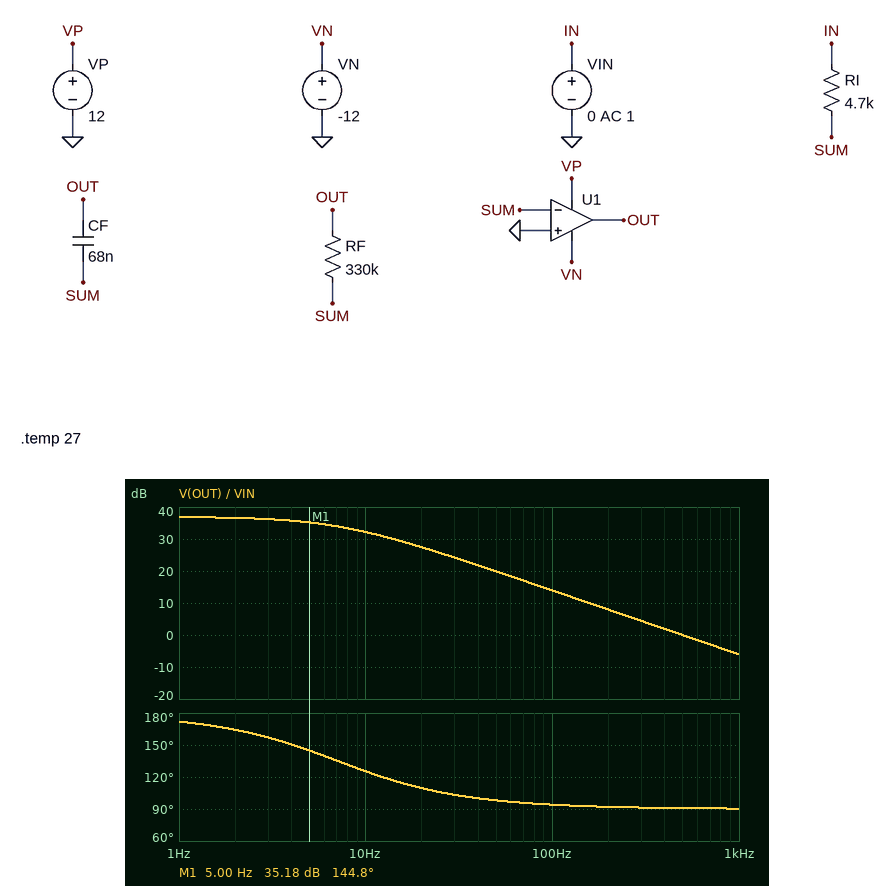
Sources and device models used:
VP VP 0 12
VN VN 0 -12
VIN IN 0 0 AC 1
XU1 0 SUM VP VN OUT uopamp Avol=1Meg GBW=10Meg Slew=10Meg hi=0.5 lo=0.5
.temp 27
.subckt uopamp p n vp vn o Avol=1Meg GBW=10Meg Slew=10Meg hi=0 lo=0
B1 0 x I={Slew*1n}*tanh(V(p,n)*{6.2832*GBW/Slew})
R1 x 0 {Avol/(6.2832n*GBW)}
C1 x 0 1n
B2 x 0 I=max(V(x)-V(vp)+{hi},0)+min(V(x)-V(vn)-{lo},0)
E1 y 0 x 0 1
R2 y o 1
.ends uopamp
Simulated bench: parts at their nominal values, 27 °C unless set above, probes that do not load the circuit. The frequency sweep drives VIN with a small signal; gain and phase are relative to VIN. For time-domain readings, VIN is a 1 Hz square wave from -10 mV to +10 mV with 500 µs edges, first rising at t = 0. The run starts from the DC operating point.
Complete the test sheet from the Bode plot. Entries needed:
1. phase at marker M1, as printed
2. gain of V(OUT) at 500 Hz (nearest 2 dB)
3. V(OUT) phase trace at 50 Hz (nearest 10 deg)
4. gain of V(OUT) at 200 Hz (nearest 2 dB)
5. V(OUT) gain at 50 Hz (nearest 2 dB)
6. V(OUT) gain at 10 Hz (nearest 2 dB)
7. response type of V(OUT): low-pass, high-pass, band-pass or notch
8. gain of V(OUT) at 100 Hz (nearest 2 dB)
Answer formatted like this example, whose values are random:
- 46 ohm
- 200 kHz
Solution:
- 144.8 deg
- 0 dB
- 100 deg
- 8 dB
- 20 dB
- 32 dB
- low-pass
- 14 dB
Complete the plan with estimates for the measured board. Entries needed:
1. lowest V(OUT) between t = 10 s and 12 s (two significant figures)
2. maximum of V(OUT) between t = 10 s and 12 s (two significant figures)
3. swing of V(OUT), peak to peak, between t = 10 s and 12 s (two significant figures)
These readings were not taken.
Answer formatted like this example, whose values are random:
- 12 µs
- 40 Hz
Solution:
- -700 mV
- 700 mV
- 1.4 V
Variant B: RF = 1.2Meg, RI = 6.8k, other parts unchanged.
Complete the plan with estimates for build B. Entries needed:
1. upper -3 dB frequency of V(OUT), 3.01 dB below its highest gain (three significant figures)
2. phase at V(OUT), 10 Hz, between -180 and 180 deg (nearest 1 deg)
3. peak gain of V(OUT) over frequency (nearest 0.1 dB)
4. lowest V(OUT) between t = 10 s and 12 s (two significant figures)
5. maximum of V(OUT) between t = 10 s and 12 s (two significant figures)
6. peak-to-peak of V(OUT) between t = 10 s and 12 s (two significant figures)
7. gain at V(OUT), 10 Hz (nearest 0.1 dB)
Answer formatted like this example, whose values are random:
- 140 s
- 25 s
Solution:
- 1.95 Hz
- 101 deg
- 44.9 dB
- -1.8 V
- 1.8 V
- 3.5 V
- 30.6 dB
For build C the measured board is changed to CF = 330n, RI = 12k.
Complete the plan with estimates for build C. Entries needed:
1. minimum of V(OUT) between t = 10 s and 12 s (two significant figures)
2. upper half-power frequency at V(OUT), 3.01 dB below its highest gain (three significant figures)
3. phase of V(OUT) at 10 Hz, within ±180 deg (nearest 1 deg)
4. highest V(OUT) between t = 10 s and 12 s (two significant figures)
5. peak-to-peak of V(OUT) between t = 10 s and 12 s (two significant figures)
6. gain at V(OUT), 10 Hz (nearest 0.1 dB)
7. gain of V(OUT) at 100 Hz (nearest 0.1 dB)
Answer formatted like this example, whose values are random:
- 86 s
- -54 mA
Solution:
- -270 mV
- 1.46 Hz
- 98 deg
- 270 mV
- 540 mV
- 12.0 dB
- -7.9 dB
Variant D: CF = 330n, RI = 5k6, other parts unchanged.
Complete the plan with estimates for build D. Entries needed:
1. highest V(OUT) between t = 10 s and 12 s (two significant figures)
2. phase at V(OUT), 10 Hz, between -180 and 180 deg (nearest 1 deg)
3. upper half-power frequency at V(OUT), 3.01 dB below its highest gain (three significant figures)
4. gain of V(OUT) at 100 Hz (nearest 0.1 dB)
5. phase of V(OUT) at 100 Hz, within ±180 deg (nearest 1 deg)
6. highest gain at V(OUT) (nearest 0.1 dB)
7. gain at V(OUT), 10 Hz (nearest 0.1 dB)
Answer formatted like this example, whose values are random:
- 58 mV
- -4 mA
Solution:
- 580 mV
- 98 deg
- 1.46 Hz
- -1.3 dB
- 91 deg
- 35.4 dB
- 18.6 dB
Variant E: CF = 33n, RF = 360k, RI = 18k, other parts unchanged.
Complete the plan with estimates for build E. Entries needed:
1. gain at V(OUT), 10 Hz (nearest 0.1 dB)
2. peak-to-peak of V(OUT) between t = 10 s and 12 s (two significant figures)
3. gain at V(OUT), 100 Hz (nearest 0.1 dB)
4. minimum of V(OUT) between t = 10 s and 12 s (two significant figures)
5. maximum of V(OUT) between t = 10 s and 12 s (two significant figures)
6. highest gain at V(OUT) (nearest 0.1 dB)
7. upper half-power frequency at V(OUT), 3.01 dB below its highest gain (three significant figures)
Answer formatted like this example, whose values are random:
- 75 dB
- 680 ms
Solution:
- 24.1 dB
- 400 mV
- 8.5 dB
- -200 mV
- 200 mV
- 26.0 dB
- 13.4 Hz
